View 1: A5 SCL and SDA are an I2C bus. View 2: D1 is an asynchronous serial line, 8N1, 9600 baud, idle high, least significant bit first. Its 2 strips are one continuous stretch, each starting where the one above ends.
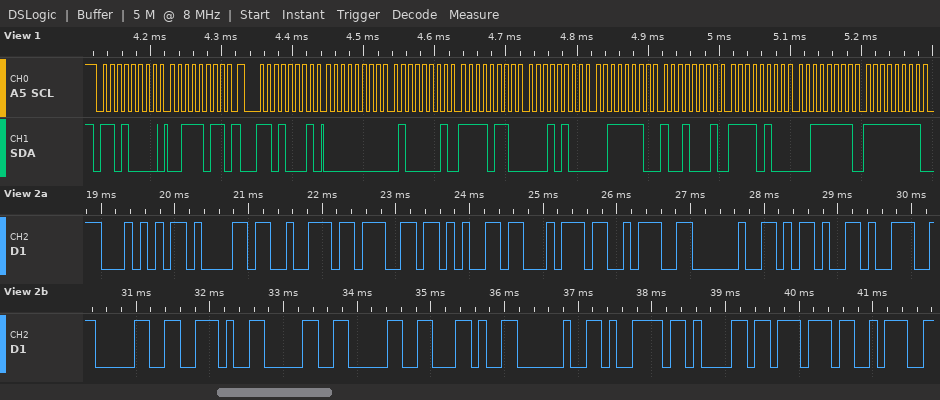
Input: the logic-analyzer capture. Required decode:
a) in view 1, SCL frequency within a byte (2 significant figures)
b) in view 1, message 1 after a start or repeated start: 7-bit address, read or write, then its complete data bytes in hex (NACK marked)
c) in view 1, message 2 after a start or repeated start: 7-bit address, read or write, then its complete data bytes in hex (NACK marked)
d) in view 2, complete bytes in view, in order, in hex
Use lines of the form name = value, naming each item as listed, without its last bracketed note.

in view 1, SCL frequency within a byte = 100 kHz
in view 1, message 1 after a start or repeated start: 7-bit address, read or write, then its complete data bytes in hex = 0x68 write: 3B
in view 1, message 2 after a start or repeated start: 7-bit address, read or write, then its complete data bytes in hex = 0x68 read: 00 41 F6 14 3E 91 F4 3F FF
in view 2, complete bytes in view, in order, in hex = 54 61 72 67 65 74 3A 20 2D 39 30 2E 30 30 2C 20 79 61 77 3A
